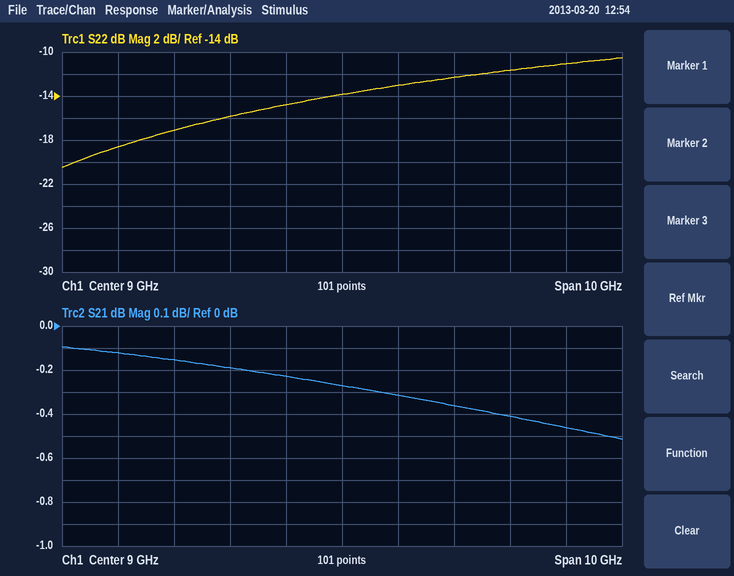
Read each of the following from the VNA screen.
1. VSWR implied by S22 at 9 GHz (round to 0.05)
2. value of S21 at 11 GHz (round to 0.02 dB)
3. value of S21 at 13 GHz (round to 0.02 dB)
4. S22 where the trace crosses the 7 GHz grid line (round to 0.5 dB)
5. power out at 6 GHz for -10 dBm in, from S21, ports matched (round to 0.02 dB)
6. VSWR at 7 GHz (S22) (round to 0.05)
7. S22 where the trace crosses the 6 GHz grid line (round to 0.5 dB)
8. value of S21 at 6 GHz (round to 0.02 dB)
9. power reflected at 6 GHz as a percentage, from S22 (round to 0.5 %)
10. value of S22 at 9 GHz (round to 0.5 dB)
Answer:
1.50
-0.36 dB
-0.46 dB
-16.0 dB
-10.16 dBm
1.40
-17.0 dB
-0.16 dB
2.0 %
-14.0 dB
